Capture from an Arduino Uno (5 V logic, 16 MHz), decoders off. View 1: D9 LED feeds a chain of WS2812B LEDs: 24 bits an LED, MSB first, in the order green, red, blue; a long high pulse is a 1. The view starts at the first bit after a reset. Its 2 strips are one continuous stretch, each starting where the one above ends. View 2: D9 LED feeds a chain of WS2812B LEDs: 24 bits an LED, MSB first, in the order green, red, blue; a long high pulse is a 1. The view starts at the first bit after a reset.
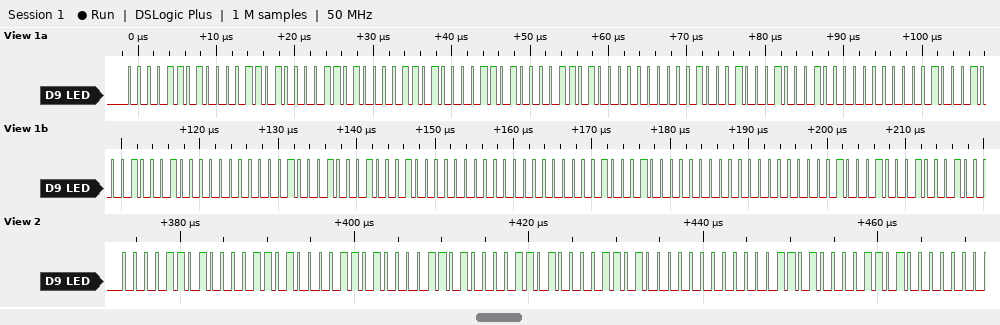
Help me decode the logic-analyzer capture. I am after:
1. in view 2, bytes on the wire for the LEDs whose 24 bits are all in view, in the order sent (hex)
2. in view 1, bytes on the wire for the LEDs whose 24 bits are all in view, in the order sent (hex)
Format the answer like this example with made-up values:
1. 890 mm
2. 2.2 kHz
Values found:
1. 0D 0D 0D 0D 0D 0D 00 0D 0D
2. 0D 0D 0D 0D 0D 0D 00 22 22 00 22 22 00 22 22 00 00 22 00 00 22
